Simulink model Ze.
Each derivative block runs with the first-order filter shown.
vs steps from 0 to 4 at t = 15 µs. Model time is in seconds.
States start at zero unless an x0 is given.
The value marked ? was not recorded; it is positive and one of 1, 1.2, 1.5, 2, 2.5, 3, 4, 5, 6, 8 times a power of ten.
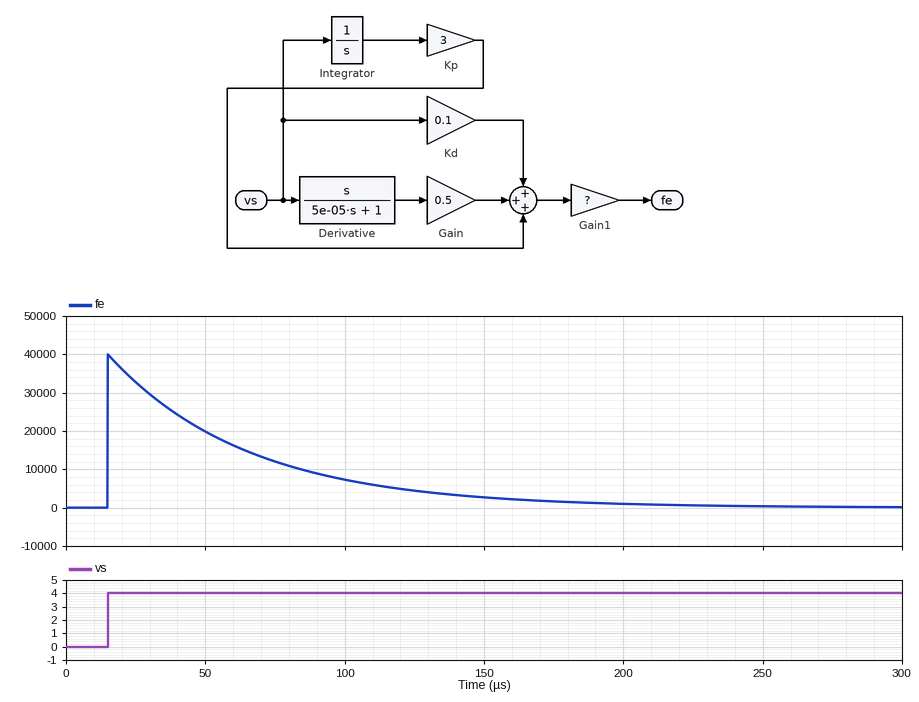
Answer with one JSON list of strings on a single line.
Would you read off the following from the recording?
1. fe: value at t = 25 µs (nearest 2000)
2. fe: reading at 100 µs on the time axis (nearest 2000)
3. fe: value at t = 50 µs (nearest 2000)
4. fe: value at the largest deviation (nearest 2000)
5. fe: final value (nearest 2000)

["32000", "8000", "20000", "40000", "0"]
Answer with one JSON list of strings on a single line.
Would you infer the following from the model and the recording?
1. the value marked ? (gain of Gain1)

["1"]
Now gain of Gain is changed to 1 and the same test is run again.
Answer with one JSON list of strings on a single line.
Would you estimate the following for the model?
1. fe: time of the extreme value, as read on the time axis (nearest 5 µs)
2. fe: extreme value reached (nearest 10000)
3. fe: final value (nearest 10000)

["15 µs", "80000", "0"]
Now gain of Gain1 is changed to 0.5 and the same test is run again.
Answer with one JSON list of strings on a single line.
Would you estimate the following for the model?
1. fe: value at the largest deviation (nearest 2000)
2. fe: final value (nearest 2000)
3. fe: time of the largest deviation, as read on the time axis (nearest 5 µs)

["20000", "0", "15 µs"]
